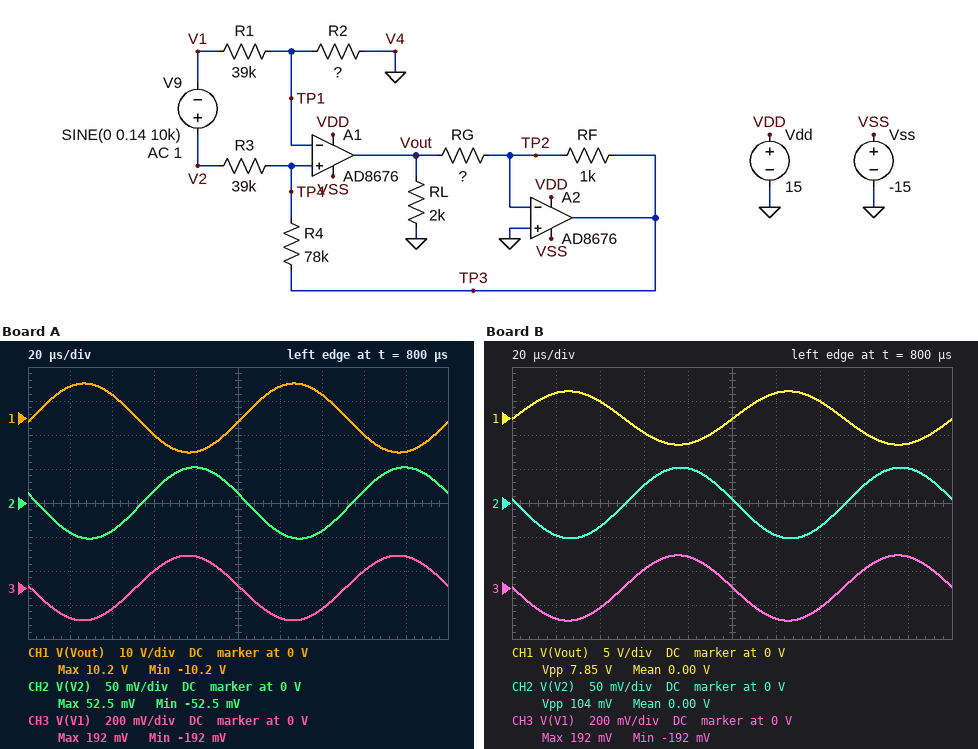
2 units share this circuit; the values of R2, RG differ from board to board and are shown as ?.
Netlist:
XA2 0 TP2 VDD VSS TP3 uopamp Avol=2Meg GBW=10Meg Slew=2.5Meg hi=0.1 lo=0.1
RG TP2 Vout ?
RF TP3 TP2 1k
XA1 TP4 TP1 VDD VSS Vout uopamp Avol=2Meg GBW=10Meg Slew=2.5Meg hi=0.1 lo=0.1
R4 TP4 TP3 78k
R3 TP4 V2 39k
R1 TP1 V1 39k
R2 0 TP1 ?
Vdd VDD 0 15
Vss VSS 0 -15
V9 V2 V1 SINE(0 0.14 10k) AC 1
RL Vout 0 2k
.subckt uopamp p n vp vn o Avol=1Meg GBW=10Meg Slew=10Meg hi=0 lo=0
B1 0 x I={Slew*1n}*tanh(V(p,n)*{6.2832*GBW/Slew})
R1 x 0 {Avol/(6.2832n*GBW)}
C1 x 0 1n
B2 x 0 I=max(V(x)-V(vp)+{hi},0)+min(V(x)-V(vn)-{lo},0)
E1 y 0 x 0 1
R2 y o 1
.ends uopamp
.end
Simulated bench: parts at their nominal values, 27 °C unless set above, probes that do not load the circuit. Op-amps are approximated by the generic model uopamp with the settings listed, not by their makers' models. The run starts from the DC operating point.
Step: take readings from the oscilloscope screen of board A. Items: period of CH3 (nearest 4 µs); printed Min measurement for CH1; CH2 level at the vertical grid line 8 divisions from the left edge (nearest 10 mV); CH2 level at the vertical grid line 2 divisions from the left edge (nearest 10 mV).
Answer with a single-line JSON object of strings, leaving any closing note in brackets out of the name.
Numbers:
{"period of CH3": "100 µs", "printed Min measurement for CH1": "-10.2 V", "CH2 level at the vertical grid line 8 divisions from the left edge": "20 mV", "CH2 level at the vertical grid line 2 divisions from the left edge": "-40 mV"}
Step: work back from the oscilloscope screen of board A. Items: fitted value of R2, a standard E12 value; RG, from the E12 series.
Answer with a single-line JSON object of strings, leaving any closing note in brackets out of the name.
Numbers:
{"fitted value of R2, a standard E12 value": "68 kΩ", "RG, from the E12 series": "39 kΩ"}
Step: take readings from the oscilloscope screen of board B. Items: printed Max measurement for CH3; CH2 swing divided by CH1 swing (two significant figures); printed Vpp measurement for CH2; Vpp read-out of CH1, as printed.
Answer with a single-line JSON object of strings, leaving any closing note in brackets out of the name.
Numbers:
{"printed Max measurement for CH3": "192 mV", "CH2 swing divided by CH1 swing": "0.013", "printed Vpp measurement for CH2": "104 mV", "Vpp read-out of CH1, as printed": "7.85 V"}
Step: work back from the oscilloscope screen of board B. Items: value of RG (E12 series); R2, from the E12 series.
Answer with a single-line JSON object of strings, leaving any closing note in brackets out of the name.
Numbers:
{"value of RG": "15 kΩ", "R2, from the E12 series": "68 kΩ"}
